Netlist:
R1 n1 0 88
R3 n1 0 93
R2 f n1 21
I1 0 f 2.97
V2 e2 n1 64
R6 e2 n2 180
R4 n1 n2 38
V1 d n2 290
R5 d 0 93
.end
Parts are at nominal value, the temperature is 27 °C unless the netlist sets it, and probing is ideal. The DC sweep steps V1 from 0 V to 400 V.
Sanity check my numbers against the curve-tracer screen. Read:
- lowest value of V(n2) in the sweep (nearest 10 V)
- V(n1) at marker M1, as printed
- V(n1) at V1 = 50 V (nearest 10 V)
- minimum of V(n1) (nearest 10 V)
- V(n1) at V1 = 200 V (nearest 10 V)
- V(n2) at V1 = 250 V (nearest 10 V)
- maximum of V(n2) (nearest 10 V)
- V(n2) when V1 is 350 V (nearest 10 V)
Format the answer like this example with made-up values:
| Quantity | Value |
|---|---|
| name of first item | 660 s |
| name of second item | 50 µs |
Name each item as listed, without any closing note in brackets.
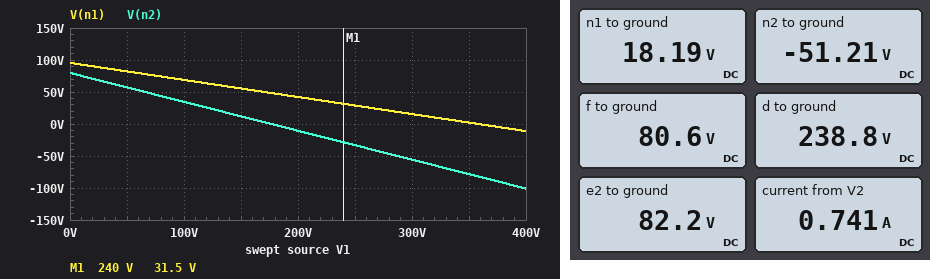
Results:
| Quantity | Value |
|---|---|
| lowest value of V(n2) in the sweep | -100 V |
| V(n1) at marker M1, as printed | 31.5 V |
| V(n1) at V1 = 50 V | 80 V |
| minimum of V(n1) | -10 V |
| V(n1) at V1 = 200 V | 40 V |
| V(n2) at V1 = 250 V | -30 V |
| maximum of V(n2) | 80 V |
| V(n2) when V1 is 350 V | -80 V |
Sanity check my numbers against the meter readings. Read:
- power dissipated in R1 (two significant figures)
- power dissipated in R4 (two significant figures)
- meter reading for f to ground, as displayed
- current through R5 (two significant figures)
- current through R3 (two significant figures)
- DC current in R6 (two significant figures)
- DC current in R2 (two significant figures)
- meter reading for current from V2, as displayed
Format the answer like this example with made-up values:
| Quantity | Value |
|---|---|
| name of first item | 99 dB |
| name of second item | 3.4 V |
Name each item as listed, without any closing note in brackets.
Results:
| Quantity | Value |
|---|---|
| power dissipated in R1 | 3.8 W |
| power dissipated in R4 | 130 W |
| meter reading for f to ground, as displayed | 80.6 V |
| current through R5 | 2.6 A |
| current through R3 | 200 mA |
| DC current in R6 | 740 mA |
| DC current in R2 | 3.0 A |
| meter reading for current from V2, as displayed | 0.741 A |
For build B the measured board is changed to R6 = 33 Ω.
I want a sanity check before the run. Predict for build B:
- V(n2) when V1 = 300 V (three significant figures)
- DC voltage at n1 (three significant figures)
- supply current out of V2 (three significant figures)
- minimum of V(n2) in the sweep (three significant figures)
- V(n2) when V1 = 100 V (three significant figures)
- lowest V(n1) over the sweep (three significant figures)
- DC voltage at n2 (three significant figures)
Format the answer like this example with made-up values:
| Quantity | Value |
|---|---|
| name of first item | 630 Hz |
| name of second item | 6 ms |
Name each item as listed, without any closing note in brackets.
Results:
| Quantity | Value |
|---|---|
| V(n2) when V1 = 300 V | -20.5 V |
| DC voltage at n1 | 1.28 V |
| supply current out of V2 | 2.48 A |
| minimum of V(n2) in the sweep | -60.8 V |
| V(n2) when V1 = 100 V | 60.2 V |
| lowest V(n1) over the sweep | -30.6 V |
| DC voltage at n2 | -16.4 V |
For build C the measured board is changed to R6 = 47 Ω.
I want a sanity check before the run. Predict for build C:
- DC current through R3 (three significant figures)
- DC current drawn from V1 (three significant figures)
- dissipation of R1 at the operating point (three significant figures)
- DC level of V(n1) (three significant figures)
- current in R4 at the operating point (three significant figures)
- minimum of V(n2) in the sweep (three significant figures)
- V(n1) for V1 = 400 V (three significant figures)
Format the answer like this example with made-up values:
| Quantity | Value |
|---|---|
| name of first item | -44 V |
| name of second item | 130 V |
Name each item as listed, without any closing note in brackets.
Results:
| Quantity | Value |
|---|---|
| DC current through R3 | 61.1 mA |
| DC current drawn from V1 | 2.84 A |
| dissipation of R1 at the operating point | 367 mW |
| DC level of V(n1) | 5.68 V |
| current in R4 at the operating point | 820 mA |
| minimum of V(n2) in the sweep | -71.2 V |
| V(n1) for V1 = 400 V | -25.6 V |
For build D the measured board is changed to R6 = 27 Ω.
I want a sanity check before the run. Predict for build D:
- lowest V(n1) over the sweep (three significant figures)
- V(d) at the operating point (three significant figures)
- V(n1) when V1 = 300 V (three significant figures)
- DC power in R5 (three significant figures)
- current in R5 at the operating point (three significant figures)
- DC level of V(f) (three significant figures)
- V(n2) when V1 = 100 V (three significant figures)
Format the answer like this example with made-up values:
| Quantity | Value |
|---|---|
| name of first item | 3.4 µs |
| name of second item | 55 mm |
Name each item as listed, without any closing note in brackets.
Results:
| Quantity | Value |
|---|---|
| lowest V(n1) over the sweep | -33.6 V |
| V(d) at the operating point | 279 V |
| V(n1) when V1 = 300 V | -4.21 V |
| DC power in R5 | 836 W |
| current in R5 at the operating point | 3.00 A |
| DC level of V(f) | 61.1 V |
| V(n2) when V1 = 100 V | 64.1 V |
